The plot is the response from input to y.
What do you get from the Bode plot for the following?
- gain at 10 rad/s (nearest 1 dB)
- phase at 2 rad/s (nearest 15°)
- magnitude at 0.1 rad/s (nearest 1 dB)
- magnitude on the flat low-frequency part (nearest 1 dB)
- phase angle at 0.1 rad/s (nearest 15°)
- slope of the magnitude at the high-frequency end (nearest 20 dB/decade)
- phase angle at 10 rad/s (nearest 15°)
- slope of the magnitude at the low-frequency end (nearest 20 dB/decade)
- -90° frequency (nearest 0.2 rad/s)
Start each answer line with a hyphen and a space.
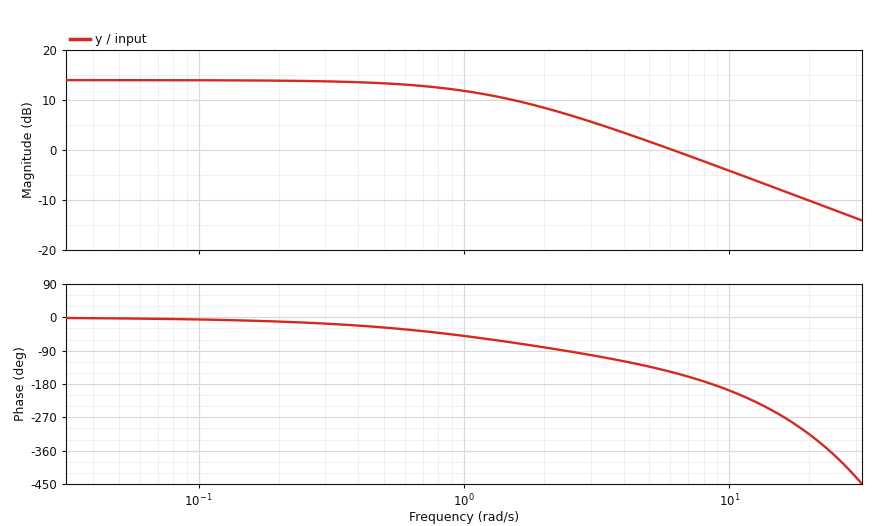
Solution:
- -4 dB
- -75°
- 14 dB
- 14 dB
- 0°
- -20 dB/decade
- -195°
- 0 dB/decade
- 2.4 rad/s
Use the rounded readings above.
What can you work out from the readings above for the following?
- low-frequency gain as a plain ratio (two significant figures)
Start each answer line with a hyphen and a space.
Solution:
- 5.0
